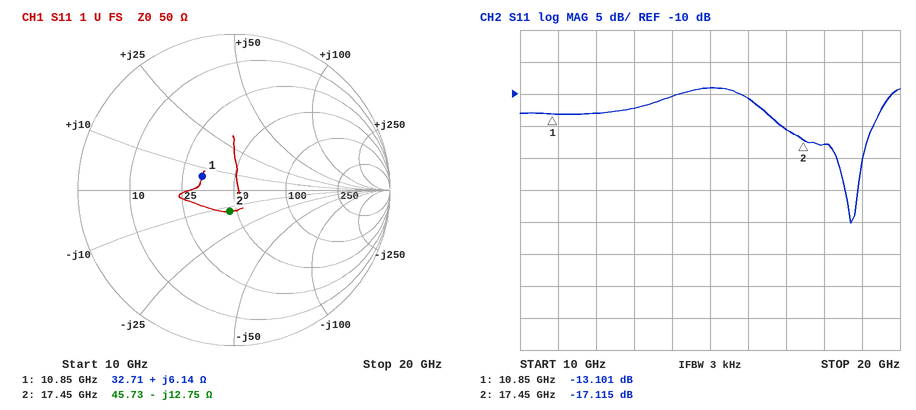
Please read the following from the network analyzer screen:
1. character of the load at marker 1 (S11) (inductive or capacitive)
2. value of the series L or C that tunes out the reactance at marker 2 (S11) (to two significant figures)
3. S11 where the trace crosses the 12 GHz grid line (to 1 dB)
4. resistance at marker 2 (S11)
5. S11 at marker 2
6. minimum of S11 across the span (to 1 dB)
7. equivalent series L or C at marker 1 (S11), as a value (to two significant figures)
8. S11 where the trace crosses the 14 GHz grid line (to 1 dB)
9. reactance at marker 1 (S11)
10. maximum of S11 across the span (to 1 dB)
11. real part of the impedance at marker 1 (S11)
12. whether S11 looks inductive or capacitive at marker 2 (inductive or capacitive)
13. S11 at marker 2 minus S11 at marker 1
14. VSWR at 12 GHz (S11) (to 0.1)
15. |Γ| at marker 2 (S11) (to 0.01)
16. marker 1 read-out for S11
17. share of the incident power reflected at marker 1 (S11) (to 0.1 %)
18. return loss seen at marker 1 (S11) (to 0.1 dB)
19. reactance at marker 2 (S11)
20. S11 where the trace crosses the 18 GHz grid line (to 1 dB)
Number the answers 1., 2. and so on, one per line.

1. inductive
2. 120 pH
3. -13 dB
4. 45.73 Ω
5. -17.115 dB
6. -30 dB
7. 90 pH
8. -10 dB
9. +6.14 Ω
10. -9 dB
11. 32.71 Ω
12. capacitive
13. -4.014 dB
14. 1.6
15. 0.14
16. -13.101 dB
17. 4.9 %
18. 13.1 dB
19. -12.75 Ω
20. -18 dB
